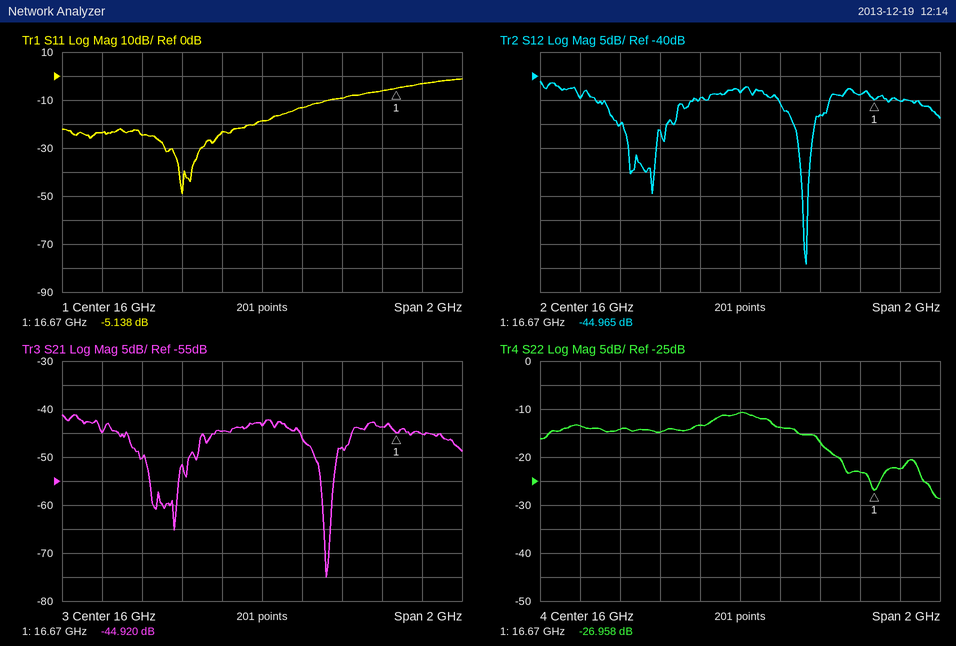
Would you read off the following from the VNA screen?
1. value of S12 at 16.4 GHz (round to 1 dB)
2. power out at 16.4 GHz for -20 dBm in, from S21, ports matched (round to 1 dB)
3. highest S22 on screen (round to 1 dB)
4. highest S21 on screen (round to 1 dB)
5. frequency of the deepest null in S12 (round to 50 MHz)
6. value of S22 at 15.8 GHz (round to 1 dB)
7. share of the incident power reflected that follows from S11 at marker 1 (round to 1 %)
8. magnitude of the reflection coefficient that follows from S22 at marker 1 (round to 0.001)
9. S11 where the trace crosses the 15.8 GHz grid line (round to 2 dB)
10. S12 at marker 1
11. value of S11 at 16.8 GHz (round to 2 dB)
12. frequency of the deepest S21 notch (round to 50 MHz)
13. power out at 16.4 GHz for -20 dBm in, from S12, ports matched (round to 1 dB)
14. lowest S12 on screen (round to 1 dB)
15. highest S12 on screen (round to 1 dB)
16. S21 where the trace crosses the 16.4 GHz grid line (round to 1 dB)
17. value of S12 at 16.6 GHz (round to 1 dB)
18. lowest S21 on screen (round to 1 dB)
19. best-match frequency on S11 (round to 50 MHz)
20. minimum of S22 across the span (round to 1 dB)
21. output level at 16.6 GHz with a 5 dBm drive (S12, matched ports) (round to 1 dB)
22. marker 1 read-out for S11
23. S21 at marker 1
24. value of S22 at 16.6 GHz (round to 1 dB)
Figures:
-48 dB
-68 dBm
-11 dB
-41 dB
16.35 GHz
-13 dB
31 %
0.045
-24 dB
-44.965 dB
-4 dB
16.30 GHz
-68 dBm
-79 dB
-41 dB
-48 dB
-44 dB
-75 dB
15.60 GHz
-29 dB
-39 dBm
-5.138 dB
-44.920 dB
-23 dB
